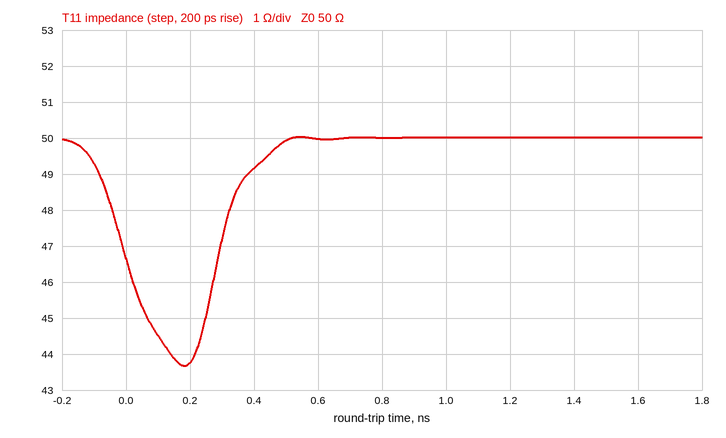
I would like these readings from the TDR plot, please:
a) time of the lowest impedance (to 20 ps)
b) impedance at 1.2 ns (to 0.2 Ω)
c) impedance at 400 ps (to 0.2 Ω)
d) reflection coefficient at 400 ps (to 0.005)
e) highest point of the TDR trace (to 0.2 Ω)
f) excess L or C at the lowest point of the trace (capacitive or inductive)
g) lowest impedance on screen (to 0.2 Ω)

180 ps
50.0 Ω
49.2 Ω
-0.010
50.0 Ω
capacitive
43.6 Ω
